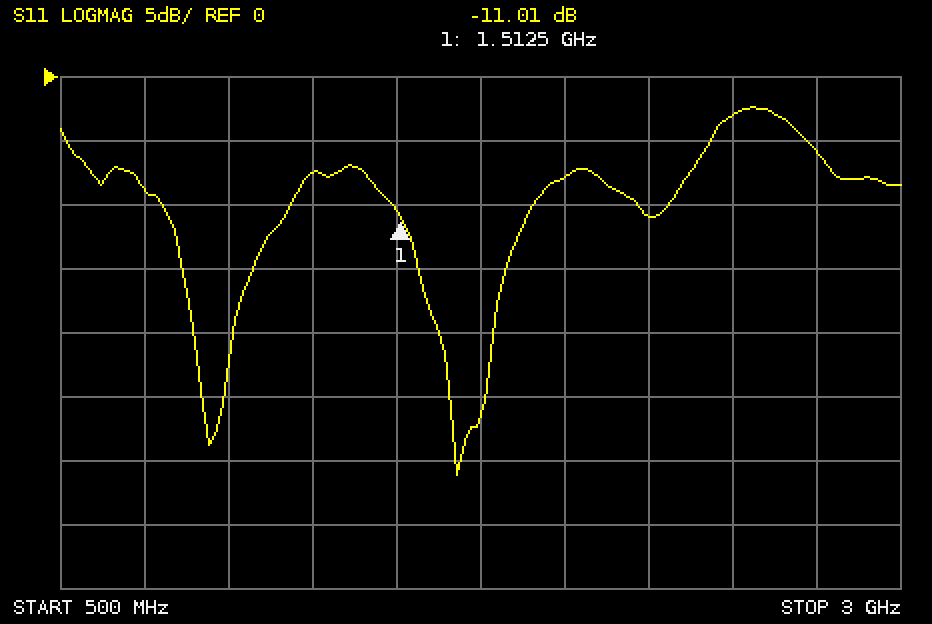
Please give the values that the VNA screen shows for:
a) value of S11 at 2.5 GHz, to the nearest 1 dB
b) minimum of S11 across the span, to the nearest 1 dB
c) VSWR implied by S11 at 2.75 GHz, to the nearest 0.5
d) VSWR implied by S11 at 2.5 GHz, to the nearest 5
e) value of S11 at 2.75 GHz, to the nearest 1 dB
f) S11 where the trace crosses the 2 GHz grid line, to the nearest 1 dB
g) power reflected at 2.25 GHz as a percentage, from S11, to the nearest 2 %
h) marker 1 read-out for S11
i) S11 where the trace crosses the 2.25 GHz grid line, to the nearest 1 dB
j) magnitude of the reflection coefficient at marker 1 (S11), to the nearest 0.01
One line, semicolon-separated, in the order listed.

-3 dB; -31 dB; 3.0; 5; -6 dB; -8 dB; 8 %; -11.01 dB; -11 dB; 0.28
